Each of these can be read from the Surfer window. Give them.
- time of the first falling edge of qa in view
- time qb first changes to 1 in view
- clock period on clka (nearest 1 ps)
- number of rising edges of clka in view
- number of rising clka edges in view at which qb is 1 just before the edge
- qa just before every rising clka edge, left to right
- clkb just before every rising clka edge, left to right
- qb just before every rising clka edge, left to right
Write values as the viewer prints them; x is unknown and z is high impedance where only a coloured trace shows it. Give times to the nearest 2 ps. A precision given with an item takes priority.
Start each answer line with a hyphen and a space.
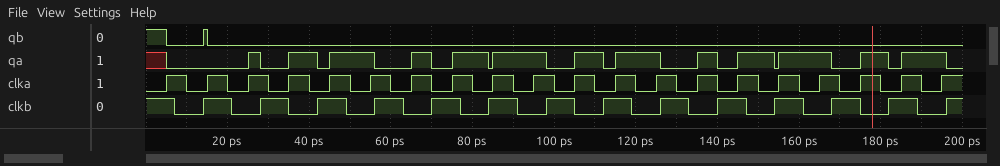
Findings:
- 28 ps
- 14 ps
- 10 ps
- 20
- 2
- x 0 0 0 0 1 0 0 0 1 0 0 1 0 0 0 1 0 0 1
- 1 1 0 1 1 0 0 1 1 0 1 1 0 0 1 1 0 1 1 0
- 1 1 0 0 0 0 0 0 0 0 0 0 0 0 0 0 0 0 0 0
